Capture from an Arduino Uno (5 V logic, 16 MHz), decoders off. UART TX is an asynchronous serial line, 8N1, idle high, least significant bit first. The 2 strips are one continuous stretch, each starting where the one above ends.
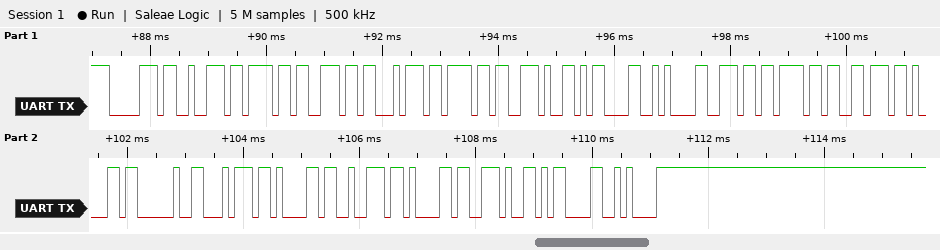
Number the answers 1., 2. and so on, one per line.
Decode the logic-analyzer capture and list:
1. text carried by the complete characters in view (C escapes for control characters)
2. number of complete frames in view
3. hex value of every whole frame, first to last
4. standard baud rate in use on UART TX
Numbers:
1. "pronto.\r\nnova tara.\r\n"
2. 21
3. 70 72 6F 6E 74 6F 2E 0D 0A 6E 6F 76 61 20 74 61 72 61 2E 0D 0A
4. 9600 baud
